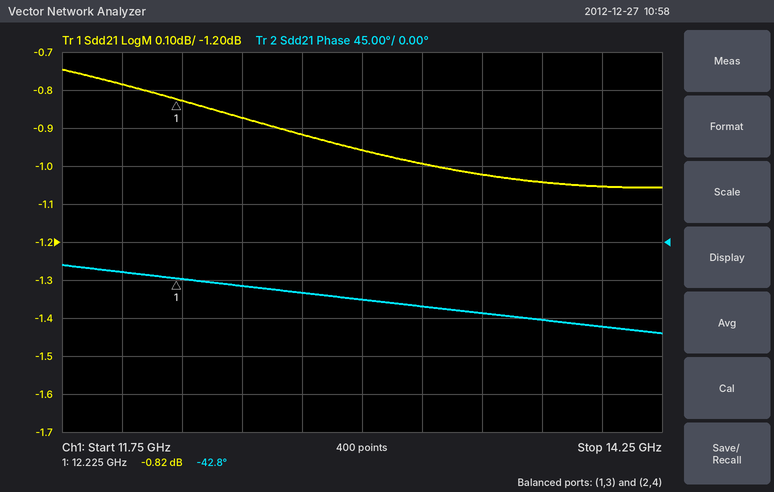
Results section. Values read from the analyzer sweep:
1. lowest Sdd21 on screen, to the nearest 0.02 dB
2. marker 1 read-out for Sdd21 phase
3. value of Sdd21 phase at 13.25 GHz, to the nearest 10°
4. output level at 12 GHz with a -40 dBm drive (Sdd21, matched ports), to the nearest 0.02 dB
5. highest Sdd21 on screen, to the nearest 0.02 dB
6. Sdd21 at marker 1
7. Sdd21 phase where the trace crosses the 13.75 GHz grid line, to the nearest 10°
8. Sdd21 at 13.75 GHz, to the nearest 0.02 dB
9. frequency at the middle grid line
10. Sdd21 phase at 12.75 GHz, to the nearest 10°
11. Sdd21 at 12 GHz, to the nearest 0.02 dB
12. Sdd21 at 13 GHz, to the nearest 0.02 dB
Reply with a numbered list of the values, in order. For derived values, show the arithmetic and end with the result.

1. -1.06 dB
2. -42.8°
3. -80°
4. -40 dBm + (-0.78 dB) = -40.78 dBm
5. -0.74 dB
6. -0.82 dB
7. -90°
8. -1.04 dB
9. 13 GHz
10. -60°
11. -0.78 dB
12. -0.96 dB
